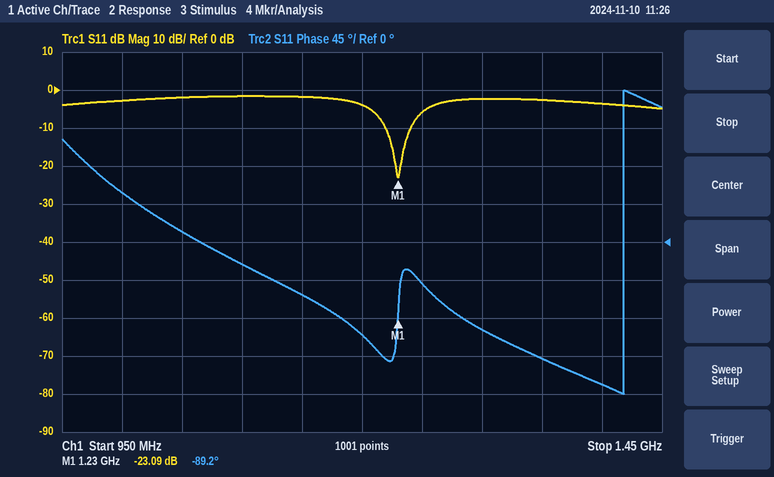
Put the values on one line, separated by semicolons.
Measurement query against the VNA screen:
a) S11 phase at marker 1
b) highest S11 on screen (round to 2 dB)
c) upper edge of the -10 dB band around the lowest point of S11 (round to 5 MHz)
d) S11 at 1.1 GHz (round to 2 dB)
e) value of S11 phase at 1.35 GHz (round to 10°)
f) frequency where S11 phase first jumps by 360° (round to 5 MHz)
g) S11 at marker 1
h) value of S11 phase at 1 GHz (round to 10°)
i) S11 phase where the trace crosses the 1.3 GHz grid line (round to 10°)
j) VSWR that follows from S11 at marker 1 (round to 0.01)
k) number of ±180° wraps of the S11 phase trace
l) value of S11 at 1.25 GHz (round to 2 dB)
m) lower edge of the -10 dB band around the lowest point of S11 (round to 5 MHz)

-89.2°; -2 dB; 1.240 GHz; -2 dB; -140°; 1.420 GHz; -23.09 dB; 60°; -100°; 1.15; 1; -6 dB; 1.220 GHz
